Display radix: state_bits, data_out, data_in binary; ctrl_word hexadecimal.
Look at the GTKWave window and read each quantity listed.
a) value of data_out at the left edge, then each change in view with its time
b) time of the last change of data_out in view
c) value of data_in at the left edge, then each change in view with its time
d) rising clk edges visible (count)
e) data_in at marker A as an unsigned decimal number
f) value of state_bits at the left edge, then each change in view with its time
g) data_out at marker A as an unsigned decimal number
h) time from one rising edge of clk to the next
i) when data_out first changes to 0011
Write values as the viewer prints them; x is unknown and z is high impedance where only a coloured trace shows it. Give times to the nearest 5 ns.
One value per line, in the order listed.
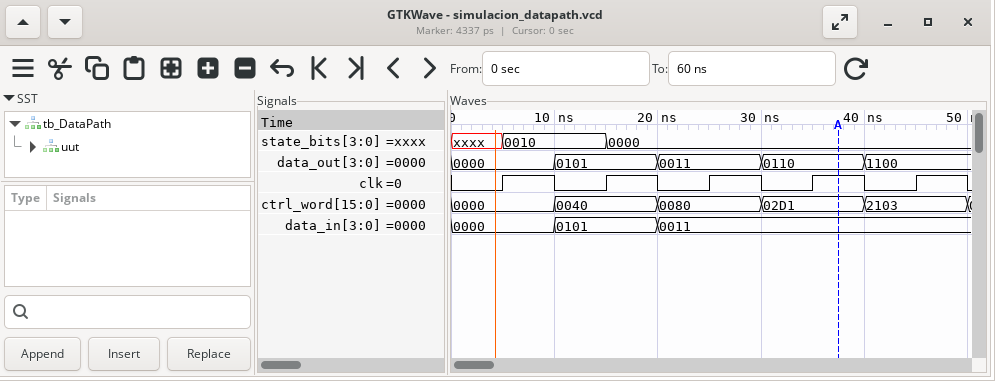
0000, 0101 at 10 ns, 0011 at 20 ns, 0110 at 30 ns, 1100 at 40 ns
40 ns
0000, 0101 at 10 ns, 0011 at 20 ns
5
3
xxxx, 0010 at 5 ns, 0000 at 15 ns
6
10 ns
20 ns
